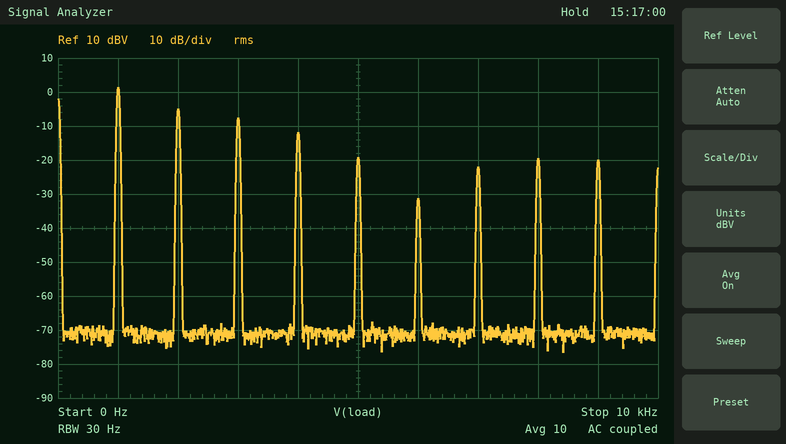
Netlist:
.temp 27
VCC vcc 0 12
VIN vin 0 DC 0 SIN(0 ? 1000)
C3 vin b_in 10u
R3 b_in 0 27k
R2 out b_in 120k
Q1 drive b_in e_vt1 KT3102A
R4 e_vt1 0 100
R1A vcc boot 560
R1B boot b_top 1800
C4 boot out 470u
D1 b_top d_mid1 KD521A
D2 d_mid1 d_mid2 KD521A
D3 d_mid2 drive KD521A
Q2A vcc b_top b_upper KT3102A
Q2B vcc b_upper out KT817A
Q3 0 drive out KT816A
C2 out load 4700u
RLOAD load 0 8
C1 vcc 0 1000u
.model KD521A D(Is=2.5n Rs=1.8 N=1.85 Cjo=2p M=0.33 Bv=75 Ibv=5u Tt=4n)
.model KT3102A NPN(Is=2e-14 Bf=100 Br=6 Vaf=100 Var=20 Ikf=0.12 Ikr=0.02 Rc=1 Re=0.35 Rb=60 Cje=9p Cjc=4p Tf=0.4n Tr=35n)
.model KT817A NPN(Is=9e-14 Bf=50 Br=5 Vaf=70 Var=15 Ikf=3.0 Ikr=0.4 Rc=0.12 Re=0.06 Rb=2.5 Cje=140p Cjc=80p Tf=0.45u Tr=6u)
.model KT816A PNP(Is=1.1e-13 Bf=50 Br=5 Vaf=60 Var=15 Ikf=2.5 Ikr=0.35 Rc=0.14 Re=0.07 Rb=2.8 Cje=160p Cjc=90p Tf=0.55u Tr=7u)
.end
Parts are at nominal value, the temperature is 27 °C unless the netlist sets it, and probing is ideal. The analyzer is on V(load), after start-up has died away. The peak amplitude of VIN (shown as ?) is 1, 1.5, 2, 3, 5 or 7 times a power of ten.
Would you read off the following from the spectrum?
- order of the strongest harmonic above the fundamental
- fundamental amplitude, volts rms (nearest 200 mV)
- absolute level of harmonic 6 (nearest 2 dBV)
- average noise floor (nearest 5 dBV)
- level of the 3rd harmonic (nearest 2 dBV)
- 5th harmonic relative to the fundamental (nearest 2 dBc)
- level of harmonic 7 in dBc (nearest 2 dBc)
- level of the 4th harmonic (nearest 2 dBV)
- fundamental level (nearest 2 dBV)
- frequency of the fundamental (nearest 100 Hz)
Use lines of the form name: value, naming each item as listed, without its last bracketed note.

order of the strongest harmonic above the fundamental: 2
fundamental amplitude, volts rms: 1.2 V
absolute level of harmonic 6: -32 dBV
average noise floor: -70 dBV
level of the 3rd harmonic: -8 dBV
5th harmonic relative to the fundamental: -20 dBc
level of harmonic 7 in dBc: -24 dBc
level of the 4th harmonic: -12 dBV
fundamental level: 2 dBV
frequency of the fundamental: 1.0 kHz
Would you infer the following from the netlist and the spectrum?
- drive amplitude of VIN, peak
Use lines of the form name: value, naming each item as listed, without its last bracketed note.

drive amplitude of VIN, peak: 200 mV
